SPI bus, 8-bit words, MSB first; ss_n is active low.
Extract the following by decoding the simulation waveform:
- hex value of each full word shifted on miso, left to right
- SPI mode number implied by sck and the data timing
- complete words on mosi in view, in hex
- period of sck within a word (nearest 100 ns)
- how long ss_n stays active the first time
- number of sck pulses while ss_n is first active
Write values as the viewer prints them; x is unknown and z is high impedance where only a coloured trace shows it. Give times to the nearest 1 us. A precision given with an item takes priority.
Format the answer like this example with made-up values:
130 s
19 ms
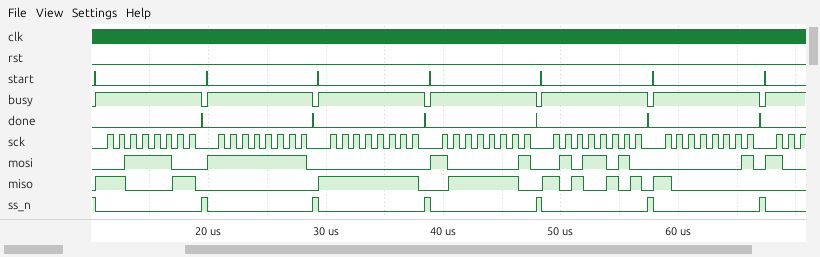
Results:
C3, 00, FF, 7E, A5, 80
0
3C, FF, 00, 81, 5A, 01
1000 ns
9 us
8
